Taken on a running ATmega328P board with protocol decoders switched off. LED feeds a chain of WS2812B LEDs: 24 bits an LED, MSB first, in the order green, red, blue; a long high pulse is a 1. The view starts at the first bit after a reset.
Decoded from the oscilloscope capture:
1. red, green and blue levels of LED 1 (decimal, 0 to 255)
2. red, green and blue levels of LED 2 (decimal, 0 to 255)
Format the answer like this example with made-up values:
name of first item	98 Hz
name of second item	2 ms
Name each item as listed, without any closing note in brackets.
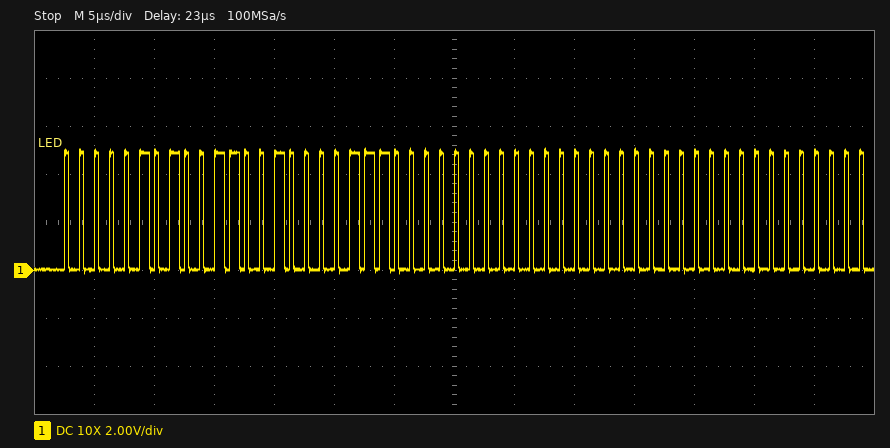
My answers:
red, green and blue levels of LED 1	50, 5, 28
red, green and blue levels of LED 2	0, 0, 0
